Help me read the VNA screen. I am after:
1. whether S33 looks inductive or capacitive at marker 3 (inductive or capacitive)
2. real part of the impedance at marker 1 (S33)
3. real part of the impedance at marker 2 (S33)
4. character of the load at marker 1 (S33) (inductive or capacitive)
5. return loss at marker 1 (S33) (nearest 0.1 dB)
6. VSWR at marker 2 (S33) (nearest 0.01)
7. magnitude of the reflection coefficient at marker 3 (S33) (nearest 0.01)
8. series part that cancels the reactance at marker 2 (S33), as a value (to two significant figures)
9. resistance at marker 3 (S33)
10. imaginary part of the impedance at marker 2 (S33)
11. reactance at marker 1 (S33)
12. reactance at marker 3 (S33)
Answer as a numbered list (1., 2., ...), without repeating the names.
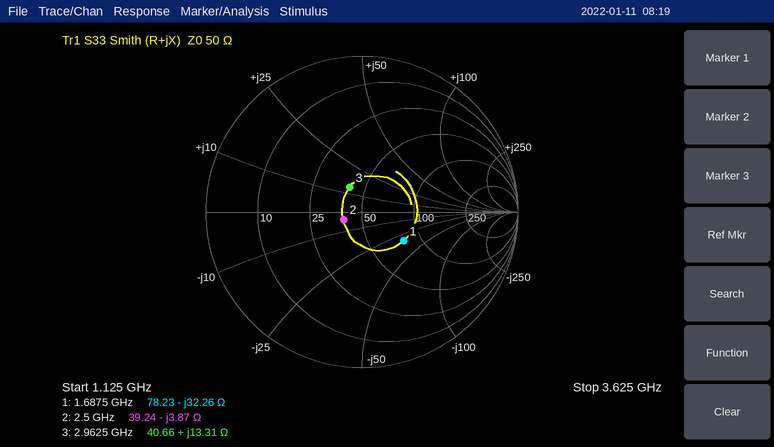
1. inductive
2. 78.23 Ω
3. 39.24 Ω
4. capacitive
5. 9.8 dB
6. 1.29
7. 0.18
8. 250 pH
9. 40.66 Ω
10. -3.87 Ω
11. -32.26 Ω
12. +13.31 Ω
